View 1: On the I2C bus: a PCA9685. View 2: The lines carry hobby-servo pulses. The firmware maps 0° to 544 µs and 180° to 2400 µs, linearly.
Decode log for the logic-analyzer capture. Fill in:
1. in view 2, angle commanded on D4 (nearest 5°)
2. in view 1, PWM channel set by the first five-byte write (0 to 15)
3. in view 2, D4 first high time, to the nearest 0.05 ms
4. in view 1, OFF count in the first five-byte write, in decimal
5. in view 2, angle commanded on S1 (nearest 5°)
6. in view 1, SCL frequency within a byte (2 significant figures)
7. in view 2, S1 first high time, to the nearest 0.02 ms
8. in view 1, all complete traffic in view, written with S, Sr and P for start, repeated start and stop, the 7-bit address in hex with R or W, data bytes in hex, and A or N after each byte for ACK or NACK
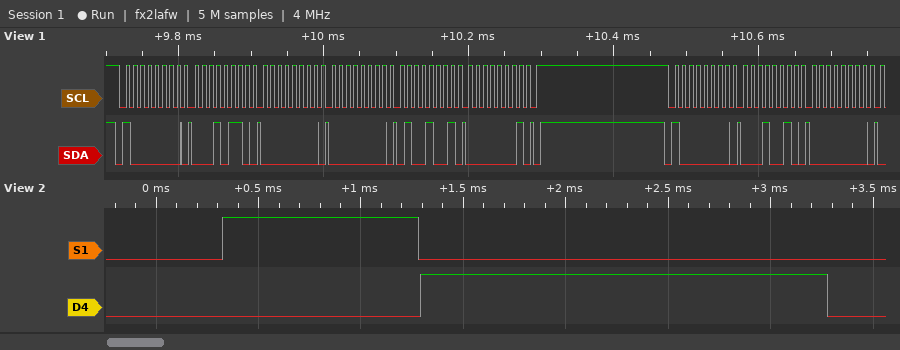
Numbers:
140°
4
2.00 ms
329
40°
100 kHz
0.96 ms
S 40W A 16 A 00 A 00 A 49 A 01 A P S 40W A 12 A 00 A
